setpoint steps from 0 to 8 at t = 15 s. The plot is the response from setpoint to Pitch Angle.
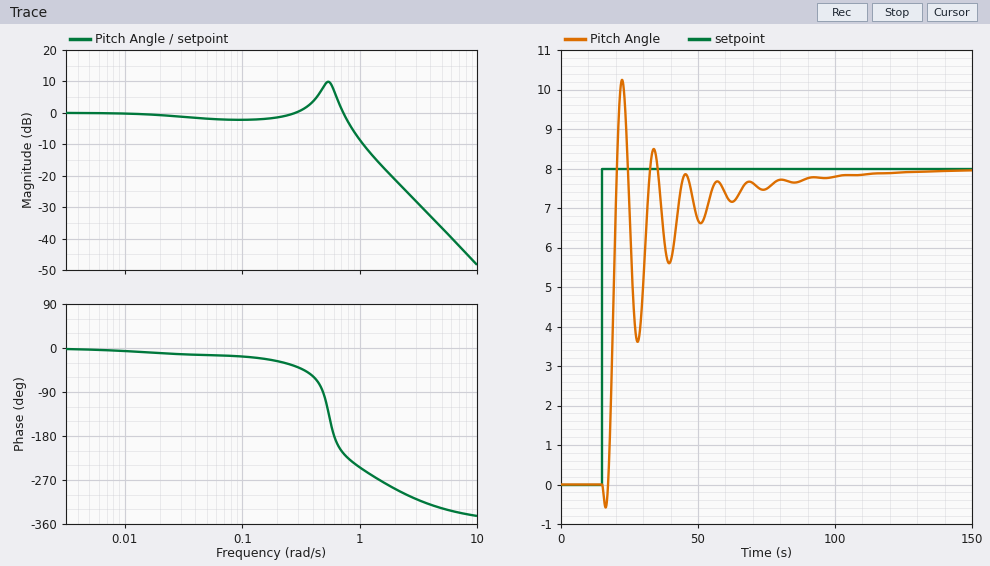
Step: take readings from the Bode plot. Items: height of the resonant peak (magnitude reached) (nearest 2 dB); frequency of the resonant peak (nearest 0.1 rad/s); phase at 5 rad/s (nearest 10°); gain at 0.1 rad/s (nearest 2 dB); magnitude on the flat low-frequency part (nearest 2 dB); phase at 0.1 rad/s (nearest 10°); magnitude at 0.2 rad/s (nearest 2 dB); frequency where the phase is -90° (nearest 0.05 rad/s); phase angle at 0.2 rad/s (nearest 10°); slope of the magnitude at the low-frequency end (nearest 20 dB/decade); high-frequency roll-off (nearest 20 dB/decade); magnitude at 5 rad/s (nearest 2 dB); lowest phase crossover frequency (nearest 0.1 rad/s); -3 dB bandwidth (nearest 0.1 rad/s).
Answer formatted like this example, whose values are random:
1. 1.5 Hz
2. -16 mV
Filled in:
1. 10 dB
2. 0.5 rad/s
3. -330°
4. -2 dB
5. 0 dB
6. -20°
7. -2 dB
8. 0.50 rad/s
9. -30°
10. 0 dB/decade
11. -40 dB/decade
12. -36 dB
13. 0.6 rad/s
14. 0.8 rad/s
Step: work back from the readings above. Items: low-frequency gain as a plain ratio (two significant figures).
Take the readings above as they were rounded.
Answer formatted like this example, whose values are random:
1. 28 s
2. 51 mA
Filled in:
1. 1.0
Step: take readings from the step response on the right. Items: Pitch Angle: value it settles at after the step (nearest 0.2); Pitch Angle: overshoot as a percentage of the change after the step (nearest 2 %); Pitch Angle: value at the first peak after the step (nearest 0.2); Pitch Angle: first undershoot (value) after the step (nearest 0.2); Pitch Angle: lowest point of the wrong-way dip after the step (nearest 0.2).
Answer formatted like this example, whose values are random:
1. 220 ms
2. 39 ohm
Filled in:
1. 8.0
2. 28 %
3. 10.2
4. 3.6
5. -0.6
